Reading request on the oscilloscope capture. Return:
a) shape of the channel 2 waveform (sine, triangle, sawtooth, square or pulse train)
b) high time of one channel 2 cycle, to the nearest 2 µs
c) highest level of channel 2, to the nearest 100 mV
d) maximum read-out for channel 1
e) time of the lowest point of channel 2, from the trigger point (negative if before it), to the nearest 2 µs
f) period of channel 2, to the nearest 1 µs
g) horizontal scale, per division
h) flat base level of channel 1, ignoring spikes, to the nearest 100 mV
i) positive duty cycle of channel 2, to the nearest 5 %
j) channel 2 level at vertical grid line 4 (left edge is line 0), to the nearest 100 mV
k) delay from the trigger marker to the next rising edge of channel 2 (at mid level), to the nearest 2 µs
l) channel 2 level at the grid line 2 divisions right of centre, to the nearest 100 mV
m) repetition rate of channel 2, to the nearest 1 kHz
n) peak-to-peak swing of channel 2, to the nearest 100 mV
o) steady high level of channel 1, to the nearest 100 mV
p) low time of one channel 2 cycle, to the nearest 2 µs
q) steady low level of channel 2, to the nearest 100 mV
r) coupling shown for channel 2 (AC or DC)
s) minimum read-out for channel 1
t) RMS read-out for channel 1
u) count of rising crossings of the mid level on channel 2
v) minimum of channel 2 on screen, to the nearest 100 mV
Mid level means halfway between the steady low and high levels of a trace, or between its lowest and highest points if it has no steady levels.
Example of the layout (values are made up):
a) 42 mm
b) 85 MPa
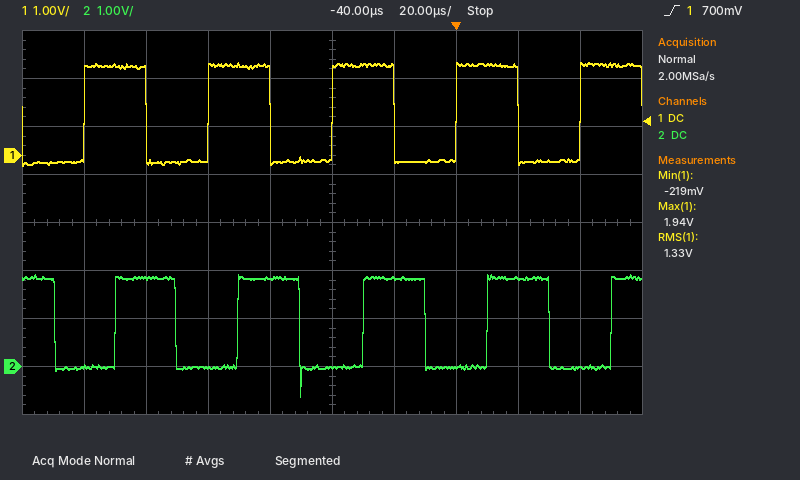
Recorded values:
a) square
b) 20 µs
c) 1.9 V
d) 1.94 V
e) -50 µs
f) 40 µs
g) 20 µs
h) -100 mV
i) 50 %
j) 1.8 V
k) 10 µs
l) 0.0 V
m) 25 kHz
n) 2.5 V
o) 1.9 V
p) 20 µs
q) 0.0 V
r) DC
s) -219 mV
t) 1.33 V
u) 5
v) -600 mV
